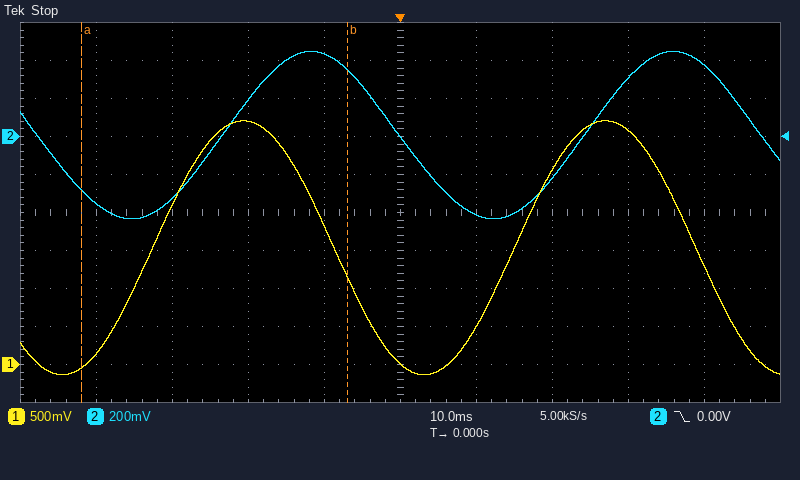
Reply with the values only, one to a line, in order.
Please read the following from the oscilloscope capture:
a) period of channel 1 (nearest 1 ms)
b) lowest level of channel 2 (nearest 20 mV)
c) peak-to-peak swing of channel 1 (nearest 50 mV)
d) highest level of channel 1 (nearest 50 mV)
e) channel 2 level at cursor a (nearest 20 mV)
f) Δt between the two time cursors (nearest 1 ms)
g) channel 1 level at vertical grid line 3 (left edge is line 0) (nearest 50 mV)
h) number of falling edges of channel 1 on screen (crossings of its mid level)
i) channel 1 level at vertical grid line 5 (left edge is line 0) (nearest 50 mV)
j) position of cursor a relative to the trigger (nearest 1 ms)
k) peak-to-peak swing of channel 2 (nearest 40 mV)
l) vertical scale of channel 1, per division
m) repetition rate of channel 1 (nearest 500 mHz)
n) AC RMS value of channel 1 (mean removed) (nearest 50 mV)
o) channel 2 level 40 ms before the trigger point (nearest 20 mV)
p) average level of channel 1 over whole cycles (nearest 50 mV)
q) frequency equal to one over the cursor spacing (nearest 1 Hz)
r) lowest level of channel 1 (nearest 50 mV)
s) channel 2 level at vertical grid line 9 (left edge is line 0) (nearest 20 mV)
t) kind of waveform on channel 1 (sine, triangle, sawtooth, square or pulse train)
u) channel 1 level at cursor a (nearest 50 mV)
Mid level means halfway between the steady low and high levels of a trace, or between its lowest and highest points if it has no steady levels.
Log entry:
48 ms
-440 mV
3.35 V
3.20 V
-280 mV
35 ms
3.20 V
2
0 mV
-42 ms
880 mV
500 mV
21.0 Hz
1.20 V
-360 mV
1.55 V
29 Hz
-150 mV
380 mV
sine
-50 mV
